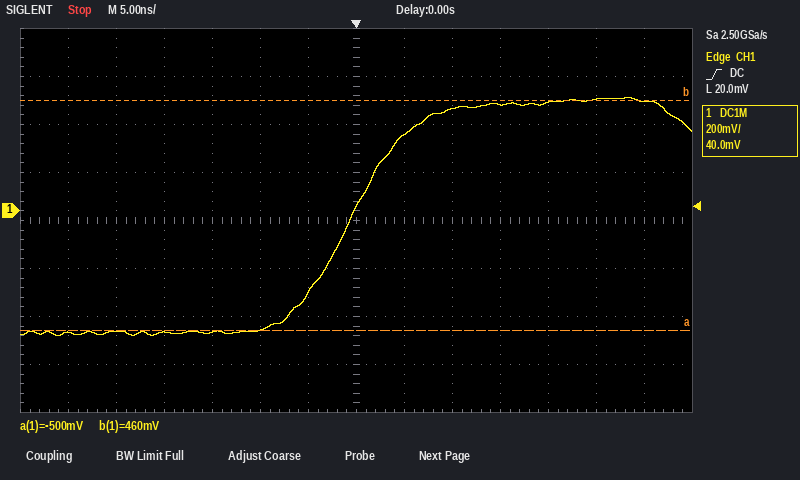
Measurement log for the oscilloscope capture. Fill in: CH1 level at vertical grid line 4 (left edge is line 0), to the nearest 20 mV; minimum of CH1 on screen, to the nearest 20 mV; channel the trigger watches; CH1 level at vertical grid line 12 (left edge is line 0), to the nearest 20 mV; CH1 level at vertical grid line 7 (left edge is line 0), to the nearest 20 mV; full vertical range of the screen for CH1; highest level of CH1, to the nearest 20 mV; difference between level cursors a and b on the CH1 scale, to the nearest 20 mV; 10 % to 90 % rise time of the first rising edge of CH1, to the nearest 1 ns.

-500 mV
-520 mV
CH1
460 mV
20 mV
1.6 V
480 mV
960 mV
13 ns
